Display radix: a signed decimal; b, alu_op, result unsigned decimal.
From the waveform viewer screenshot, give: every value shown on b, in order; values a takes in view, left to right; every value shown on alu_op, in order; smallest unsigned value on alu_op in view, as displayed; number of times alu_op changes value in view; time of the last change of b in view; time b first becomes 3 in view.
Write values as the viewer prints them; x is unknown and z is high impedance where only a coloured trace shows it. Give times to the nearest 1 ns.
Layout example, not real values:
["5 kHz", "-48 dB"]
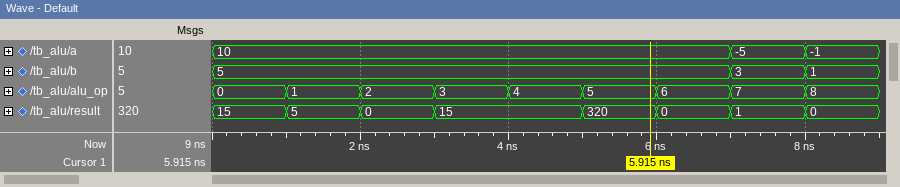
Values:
["5, 3, 1", "10, -5, -1", "0, 1, 2, 3, 4, 5, 6, 7, 8", "0", "8", "8 ns", "7 ns"]
